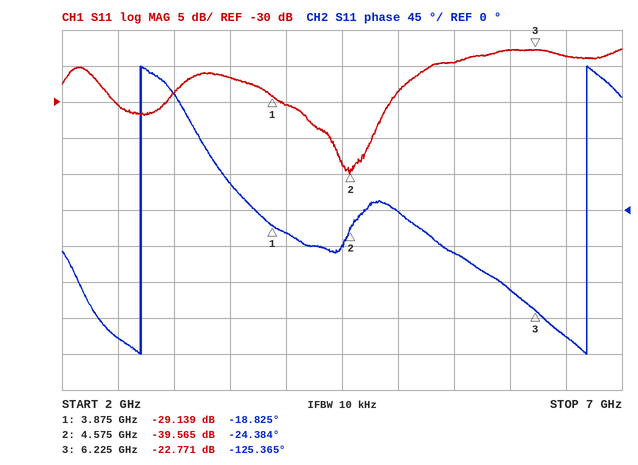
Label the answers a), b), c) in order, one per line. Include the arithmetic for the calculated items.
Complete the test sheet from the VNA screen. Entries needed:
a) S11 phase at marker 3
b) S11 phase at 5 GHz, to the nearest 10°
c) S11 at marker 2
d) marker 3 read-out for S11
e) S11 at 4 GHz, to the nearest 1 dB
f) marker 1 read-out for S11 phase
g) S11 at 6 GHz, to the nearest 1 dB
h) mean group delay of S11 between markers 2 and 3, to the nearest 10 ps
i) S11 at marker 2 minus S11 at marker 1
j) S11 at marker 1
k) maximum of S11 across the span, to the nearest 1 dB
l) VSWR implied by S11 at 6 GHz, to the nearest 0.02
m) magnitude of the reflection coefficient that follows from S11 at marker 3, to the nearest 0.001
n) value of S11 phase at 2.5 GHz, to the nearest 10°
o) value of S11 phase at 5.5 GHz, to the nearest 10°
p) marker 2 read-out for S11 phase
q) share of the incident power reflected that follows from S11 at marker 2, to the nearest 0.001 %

a) -125.365°
b) 0°
c) -39.565 dB
d) -22.771 dB
e) -30 dB
f) -18.825°
g) -23 dB
h) −(-125.365° − (-24.384°))/(360° × 1.65 GHz) ≈ 170 ps
i) -39.565 − (-29.139) = -10.426 dB
j) -29.139 dB
k) -23 dB
l) |Γ| = 10^(-23/20) = 0.0708; VSWR = (1 + 0.0708)/(1 − 0.0708) ≈ 1.15, so 1.16 to the nearest 0.02
m) 10^(-22.771/20) ≈ 0.073
n) -160°
o) -50°
p) -24.384°
q) 10^(-39.565/10) ≈ 0.011 %
